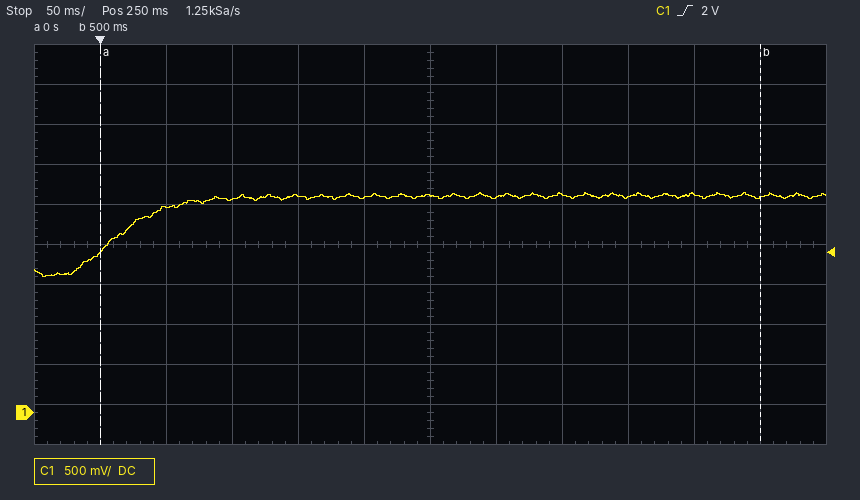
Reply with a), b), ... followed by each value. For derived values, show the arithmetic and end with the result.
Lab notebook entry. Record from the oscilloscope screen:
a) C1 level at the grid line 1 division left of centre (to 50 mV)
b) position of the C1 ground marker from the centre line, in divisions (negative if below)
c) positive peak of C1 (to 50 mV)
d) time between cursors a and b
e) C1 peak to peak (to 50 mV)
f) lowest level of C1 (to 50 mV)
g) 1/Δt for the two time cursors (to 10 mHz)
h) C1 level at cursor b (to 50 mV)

a) 2.70 V
b) -4.2 div
c) 2.75 V
d) 500 ms − (0 s) = 500 ms
e) 2.75 V − (1.70 V) = 1.05 V
f) 1.70 V
g) 1 / 500 ms ≈ 2.00 Hz
h) 2.70 V
